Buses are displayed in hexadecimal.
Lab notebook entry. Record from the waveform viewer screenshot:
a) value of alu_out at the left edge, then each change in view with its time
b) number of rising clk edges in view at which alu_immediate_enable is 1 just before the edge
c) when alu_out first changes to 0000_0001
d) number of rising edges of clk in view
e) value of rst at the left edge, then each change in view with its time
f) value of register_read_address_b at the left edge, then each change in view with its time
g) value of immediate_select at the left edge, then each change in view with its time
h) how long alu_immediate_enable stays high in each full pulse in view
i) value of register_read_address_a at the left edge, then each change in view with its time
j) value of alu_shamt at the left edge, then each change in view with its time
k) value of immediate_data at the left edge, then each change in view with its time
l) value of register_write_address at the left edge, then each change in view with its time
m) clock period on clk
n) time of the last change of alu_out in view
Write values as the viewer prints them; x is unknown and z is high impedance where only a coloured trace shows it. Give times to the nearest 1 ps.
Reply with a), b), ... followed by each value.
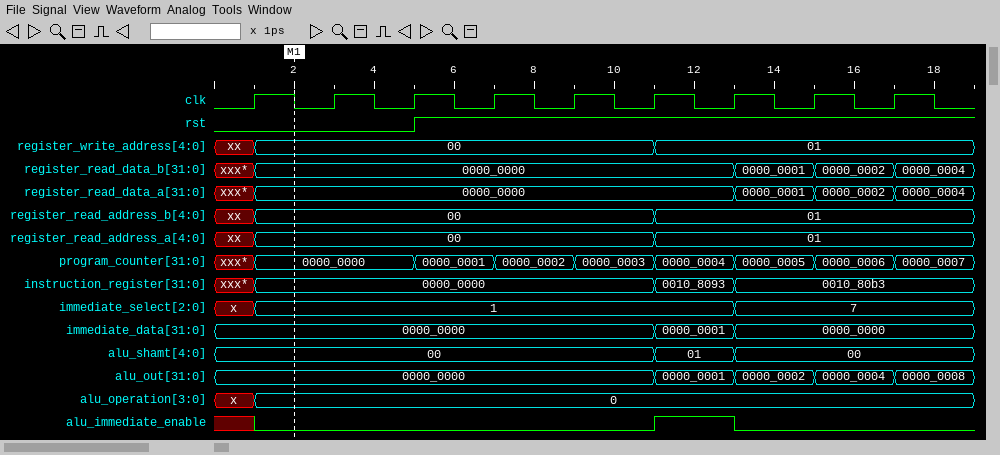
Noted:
a) 0000_0000, 0000_0001 at 11 ps, 0000_0002 at 13 ps, 0000_0004 at 15 ps, 0000_0008 at 17 ps
b) 1
c) 11 ps
d) 9
e) 0, 1 at 5 ps
f) xx, 00 at 1 ps, 01 at 11 ps
g) x, 1 at 1 ps, 7 at 13 ps
h) 2 ps
i) xx, 00 at 1 ps, 01 at 11 ps
j) 00, 01 at 11 ps, 00 at 13 ps
k) 0000_0000, 0000_0001 at 11 ps, 0000_0000 at 13 ps
l) xx, 00 at 1 ps, 01 at 11 ps
m) 2 ps
n) 17 ps
